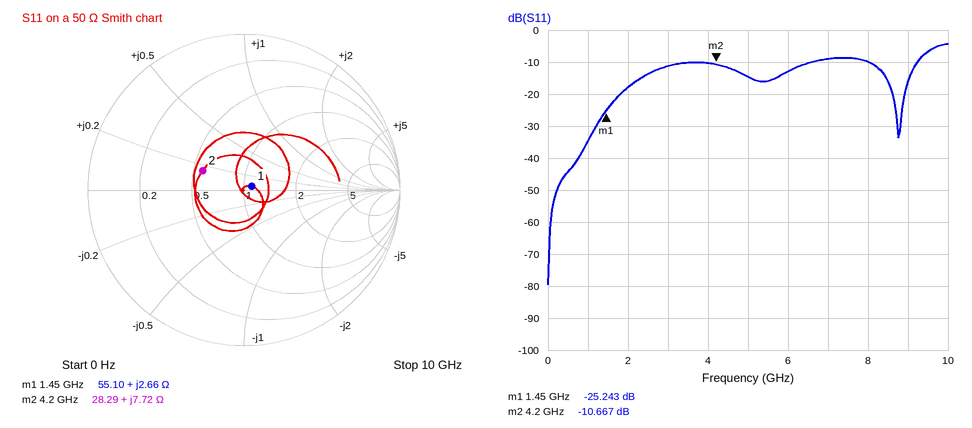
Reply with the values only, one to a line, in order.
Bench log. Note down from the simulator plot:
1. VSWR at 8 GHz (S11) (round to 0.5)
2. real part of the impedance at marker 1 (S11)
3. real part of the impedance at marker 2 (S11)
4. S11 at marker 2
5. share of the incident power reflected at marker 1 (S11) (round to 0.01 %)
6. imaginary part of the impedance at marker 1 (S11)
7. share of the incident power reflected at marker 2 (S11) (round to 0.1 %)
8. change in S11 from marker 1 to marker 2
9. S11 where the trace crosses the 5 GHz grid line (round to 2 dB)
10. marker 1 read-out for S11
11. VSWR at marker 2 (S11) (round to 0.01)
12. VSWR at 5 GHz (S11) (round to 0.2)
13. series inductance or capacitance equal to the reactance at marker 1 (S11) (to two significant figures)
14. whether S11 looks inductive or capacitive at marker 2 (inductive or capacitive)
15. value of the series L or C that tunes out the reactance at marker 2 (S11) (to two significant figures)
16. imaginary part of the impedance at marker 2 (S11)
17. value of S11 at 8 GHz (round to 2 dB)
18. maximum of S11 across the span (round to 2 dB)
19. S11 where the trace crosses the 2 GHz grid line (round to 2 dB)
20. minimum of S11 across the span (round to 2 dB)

2.0
55.10 Ω
28.29 Ω
-10.667 dB
0.30 %
+2.66 Ω
8.6 %
14.576 dB
-14 dB
-25.243 dB
1.83
1.4
290 pH
inductive
4.9 pF
+7.72 Ω
-10 dB
-4 dB
-18 dB
-80 dB
